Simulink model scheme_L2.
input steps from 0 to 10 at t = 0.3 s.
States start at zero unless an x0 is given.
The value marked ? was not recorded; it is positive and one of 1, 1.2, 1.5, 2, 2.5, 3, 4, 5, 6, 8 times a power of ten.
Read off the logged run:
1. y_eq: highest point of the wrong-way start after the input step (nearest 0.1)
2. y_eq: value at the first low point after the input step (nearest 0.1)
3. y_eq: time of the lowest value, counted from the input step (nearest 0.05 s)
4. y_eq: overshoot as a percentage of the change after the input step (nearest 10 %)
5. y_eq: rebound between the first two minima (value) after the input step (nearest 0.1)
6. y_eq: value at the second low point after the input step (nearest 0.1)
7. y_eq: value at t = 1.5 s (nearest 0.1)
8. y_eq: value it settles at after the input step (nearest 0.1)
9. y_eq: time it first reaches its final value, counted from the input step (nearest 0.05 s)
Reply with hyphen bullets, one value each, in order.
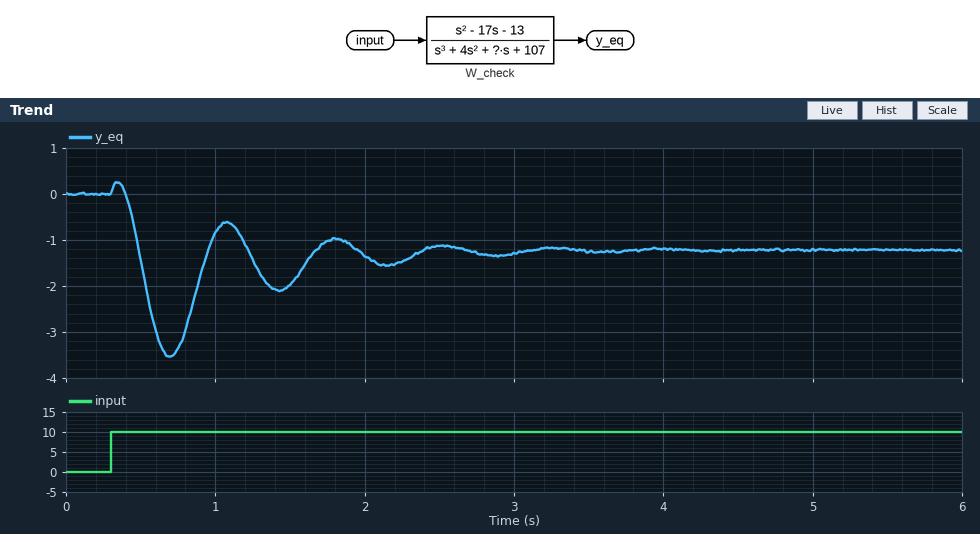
- 0.2
- -3.5
- 0.40 s
- 190 %
- -0.6
- -2.1
- -2.0
- -1.2
- 0.20 s
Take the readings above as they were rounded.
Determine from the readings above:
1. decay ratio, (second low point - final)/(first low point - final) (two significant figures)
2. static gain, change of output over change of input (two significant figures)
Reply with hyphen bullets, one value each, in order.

- 0.39
- -0.12
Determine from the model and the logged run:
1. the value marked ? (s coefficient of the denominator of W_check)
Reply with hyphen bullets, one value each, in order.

- 80
